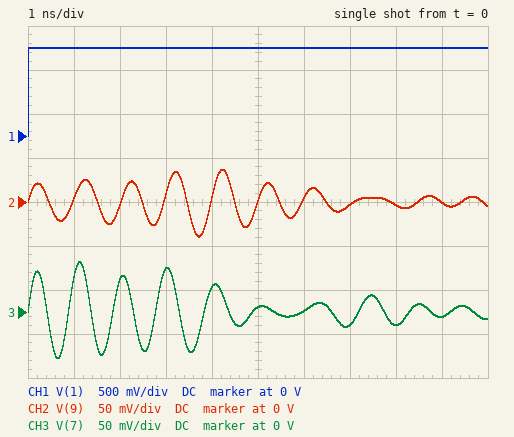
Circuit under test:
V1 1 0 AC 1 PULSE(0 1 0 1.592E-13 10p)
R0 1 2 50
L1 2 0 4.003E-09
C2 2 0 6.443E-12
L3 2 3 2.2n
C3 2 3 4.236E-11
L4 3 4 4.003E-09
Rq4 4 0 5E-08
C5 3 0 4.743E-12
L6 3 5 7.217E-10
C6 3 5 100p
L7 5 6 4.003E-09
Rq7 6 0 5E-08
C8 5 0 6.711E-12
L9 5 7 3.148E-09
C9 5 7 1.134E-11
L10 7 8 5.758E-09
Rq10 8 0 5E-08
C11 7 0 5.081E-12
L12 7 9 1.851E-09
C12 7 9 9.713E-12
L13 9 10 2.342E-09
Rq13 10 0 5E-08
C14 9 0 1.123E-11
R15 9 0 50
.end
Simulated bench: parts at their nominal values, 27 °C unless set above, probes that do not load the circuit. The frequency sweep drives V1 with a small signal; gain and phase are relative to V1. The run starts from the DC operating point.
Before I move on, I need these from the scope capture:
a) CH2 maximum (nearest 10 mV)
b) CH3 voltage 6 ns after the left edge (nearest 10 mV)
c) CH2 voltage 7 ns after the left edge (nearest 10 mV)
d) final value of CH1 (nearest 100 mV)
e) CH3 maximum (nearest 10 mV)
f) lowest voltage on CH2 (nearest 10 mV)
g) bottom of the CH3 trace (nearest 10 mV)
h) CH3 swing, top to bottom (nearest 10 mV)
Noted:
40 mV
0 V
0 V
1.0 V
60 mV
-40 mV
-50 mV
110 mV
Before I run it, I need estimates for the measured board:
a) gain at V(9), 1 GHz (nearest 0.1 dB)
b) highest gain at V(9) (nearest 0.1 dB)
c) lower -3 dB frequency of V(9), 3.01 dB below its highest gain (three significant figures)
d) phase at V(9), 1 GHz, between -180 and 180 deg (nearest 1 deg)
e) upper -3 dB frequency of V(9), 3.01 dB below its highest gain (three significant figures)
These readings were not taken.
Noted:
-6.2 dB
-6.2 dB
906 MHz
6 deg
1.10 GHz
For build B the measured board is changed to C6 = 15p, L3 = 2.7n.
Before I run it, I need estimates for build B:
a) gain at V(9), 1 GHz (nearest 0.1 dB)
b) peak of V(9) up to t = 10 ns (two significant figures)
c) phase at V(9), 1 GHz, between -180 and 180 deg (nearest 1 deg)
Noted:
-6.1 dB
41 mV
0 deg
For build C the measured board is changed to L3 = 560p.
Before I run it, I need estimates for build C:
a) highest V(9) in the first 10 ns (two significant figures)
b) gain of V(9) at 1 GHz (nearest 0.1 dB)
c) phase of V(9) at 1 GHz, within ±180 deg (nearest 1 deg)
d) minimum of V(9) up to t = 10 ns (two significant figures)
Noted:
27 mV
-7.2 dB
-19 deg
-28 mV
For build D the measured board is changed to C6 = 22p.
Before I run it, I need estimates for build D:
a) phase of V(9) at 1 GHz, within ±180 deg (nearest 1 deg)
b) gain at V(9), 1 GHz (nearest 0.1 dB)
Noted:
-2 deg
-6.1 dB
